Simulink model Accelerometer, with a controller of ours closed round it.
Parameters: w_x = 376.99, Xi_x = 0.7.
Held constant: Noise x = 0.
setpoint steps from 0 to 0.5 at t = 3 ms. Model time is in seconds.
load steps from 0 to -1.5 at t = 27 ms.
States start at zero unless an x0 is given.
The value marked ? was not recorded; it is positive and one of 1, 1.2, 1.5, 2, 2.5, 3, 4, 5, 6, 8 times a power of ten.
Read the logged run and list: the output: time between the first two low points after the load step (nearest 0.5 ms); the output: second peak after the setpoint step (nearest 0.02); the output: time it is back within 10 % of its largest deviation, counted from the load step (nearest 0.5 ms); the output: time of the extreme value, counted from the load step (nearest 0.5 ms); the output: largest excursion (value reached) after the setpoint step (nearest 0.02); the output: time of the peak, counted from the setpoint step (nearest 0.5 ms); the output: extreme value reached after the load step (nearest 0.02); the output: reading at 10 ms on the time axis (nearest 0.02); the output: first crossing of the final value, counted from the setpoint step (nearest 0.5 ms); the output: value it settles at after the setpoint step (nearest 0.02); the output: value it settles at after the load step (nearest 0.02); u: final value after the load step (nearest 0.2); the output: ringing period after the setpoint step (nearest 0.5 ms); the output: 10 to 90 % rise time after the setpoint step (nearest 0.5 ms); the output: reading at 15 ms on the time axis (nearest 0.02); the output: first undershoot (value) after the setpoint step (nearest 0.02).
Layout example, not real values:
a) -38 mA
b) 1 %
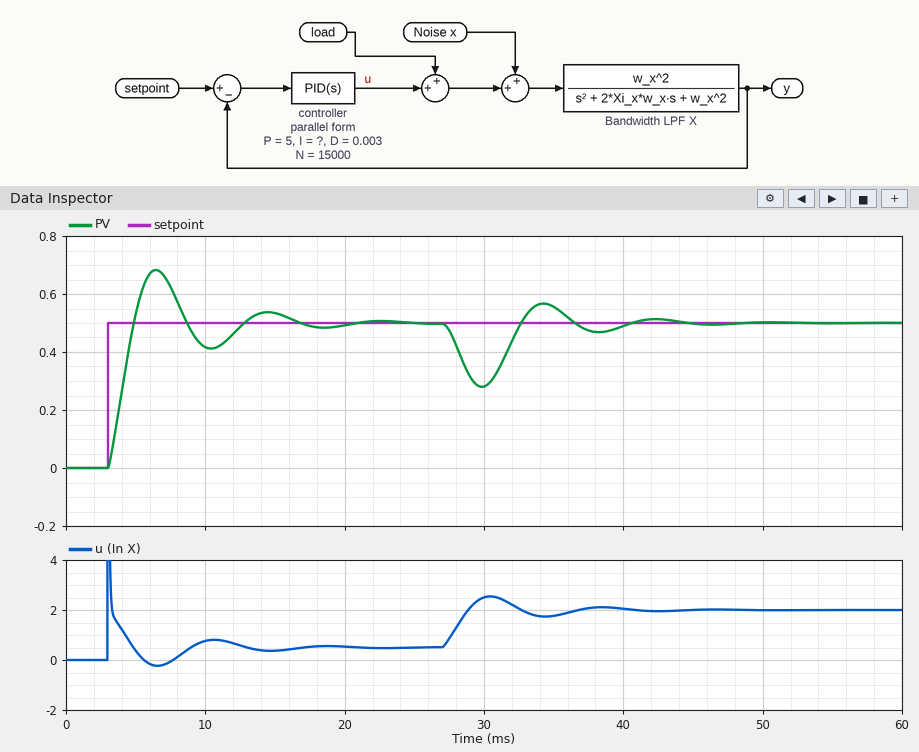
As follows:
a) 8.5 ms
b) 0.54
c) 12.5 ms
d) 3.0 ms
e) 0.68
f) 3.5 ms
g) 0.28
h) 0.42
i) 2.0 ms
j) 0.50
k) 0.50
l) 2.0
m) 8.0 ms
n) 1.5 ms
o) 0.54
p) 0.42
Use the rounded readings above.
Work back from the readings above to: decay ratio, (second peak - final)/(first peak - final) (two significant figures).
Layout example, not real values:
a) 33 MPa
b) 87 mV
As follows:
a) 0.22
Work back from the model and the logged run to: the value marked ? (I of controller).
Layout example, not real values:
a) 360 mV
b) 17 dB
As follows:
a) 2500
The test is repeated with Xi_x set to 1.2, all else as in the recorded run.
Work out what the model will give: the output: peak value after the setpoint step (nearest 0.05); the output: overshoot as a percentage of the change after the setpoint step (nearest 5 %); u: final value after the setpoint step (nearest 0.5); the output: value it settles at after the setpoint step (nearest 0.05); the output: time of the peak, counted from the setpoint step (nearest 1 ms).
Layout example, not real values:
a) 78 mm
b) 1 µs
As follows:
a) 0.65
b) 30 %
c) 0.5
d) 0.50
e) 4 ms
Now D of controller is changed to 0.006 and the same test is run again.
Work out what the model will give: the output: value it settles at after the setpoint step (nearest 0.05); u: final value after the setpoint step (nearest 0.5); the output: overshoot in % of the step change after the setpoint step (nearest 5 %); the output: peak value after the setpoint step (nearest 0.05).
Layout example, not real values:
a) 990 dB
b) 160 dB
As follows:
a) 0.50
b) 0.5
c) 20 %
d) 0.60
